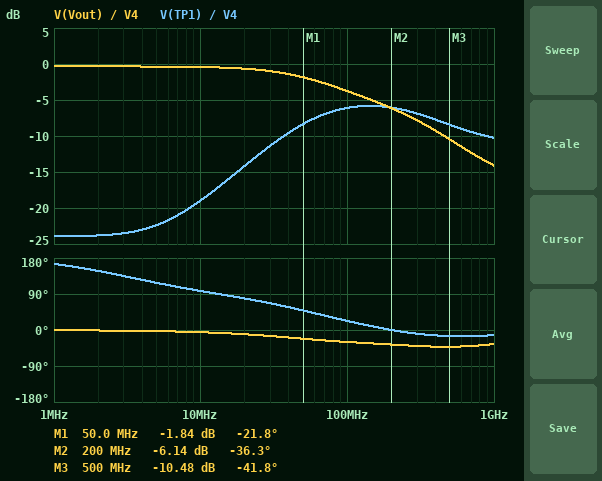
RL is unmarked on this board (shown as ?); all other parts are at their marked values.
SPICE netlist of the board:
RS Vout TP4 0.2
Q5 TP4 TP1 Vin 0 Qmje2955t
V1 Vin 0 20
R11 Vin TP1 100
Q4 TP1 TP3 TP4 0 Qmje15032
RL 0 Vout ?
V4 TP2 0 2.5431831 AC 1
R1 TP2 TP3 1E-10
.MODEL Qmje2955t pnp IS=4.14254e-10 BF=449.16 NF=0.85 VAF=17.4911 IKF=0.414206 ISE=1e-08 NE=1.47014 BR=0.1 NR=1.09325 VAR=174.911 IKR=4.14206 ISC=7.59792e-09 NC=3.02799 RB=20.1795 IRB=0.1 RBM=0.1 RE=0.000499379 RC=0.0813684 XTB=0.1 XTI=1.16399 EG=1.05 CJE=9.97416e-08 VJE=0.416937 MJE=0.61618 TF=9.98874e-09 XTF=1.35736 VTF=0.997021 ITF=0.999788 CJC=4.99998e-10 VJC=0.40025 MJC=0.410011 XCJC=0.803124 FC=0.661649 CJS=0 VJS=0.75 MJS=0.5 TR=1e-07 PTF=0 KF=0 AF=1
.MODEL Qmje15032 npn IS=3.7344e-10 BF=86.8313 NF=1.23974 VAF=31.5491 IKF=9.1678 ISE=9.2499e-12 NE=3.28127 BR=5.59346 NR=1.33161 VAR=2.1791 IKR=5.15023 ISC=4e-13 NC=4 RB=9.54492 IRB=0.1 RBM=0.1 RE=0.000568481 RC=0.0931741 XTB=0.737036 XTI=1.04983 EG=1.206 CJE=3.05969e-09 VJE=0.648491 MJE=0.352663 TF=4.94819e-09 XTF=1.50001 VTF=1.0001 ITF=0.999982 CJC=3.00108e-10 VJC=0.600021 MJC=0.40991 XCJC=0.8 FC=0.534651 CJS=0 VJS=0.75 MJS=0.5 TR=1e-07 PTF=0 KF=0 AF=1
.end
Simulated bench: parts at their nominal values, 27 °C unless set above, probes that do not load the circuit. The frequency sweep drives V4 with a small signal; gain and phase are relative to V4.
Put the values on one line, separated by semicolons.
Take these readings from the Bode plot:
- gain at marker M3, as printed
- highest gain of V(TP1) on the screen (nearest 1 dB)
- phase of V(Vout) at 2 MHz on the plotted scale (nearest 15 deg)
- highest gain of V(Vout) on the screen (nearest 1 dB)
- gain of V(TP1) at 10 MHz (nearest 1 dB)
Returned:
-10.48 dB; -6 dB; 0 deg; 0 dB; -19 dB
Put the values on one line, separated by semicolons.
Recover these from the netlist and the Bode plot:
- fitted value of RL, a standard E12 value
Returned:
270 Ω
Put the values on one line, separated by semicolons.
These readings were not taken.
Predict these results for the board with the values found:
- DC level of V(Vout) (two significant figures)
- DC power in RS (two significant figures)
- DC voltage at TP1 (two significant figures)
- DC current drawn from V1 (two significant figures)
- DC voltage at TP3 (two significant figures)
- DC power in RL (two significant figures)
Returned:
2.0 V; 11 µW; 20 V; 7.5 mA; 2.5 V; 15 mW
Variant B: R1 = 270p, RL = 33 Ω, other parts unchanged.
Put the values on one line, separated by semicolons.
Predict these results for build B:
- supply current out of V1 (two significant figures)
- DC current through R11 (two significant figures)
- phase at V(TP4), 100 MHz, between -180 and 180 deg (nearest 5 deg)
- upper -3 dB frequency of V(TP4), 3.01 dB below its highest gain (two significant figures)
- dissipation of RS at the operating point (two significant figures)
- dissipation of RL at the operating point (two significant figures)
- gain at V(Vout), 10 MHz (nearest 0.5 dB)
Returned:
61 mA; 4.1 mA; -25 deg; 34 MHz; 750 µW; 120 mW; -2.5 dB
